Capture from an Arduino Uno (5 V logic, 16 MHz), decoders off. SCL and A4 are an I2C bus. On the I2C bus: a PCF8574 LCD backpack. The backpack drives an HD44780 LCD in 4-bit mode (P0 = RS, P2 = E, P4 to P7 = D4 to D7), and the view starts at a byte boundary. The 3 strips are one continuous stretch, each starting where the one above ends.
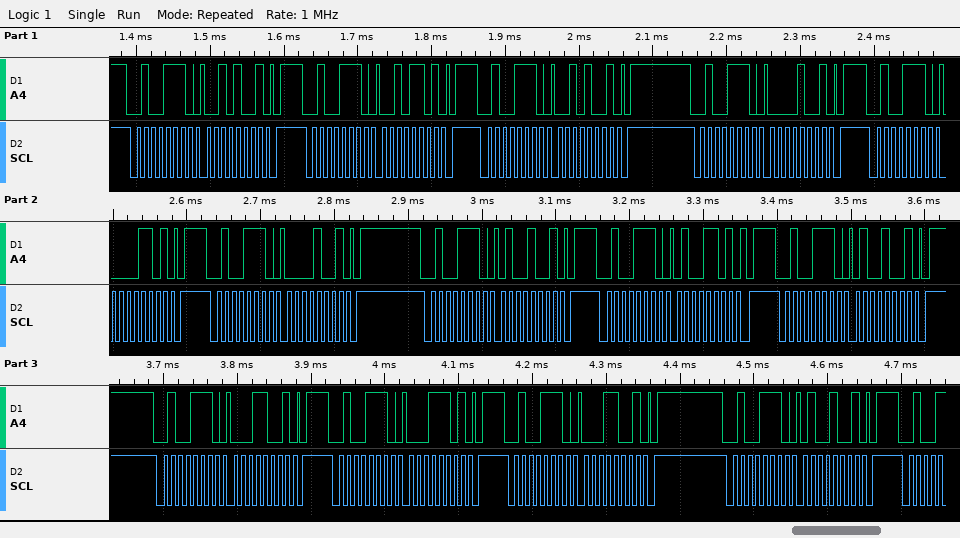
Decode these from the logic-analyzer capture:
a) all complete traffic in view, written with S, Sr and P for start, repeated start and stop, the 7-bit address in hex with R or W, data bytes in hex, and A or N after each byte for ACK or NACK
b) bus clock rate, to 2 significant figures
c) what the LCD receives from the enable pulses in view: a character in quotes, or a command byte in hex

S 27W A 29 A P S 27W A 2D A P S 27W A 29 A P S 27W A 09 A P S 27W A 0D A P S 27W A 09 A P S 27W A 49 A P S 27W A 4D A P S 27W A 49 A P S 27W A 19 A P S 27W A 1D A P S 27W A 19 A P S 27W A 49 A P
100 kHz
' ' 'A'
